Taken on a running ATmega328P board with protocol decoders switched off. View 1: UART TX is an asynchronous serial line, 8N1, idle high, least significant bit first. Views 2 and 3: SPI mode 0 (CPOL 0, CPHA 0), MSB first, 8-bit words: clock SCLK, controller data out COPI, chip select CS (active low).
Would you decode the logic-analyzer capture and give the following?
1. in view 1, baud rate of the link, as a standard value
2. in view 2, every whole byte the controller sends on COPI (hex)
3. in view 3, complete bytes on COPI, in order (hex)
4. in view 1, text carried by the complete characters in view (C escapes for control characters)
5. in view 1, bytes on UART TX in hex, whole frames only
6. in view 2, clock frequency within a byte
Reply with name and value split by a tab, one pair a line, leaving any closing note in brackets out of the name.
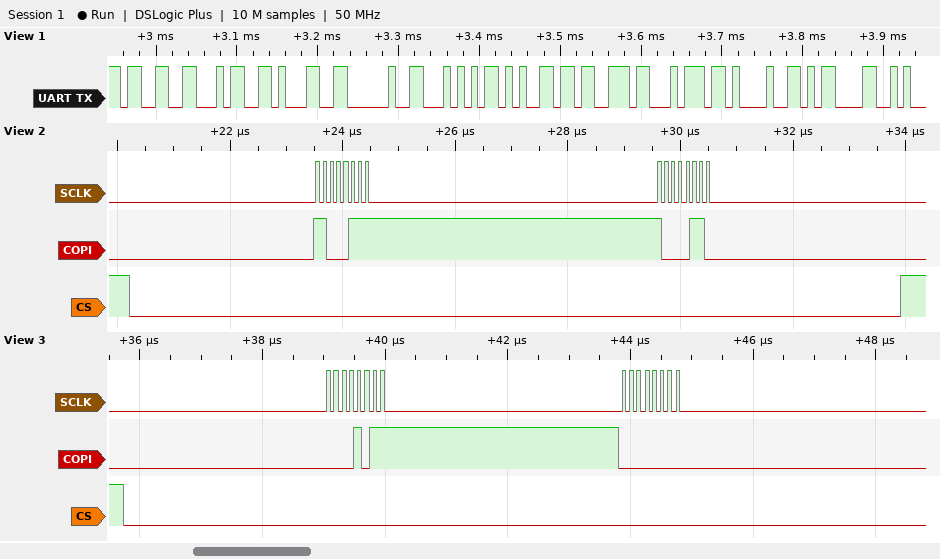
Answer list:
in view 1, baud rate of the link, as a standard value	115200 baud
in view 2, every whole byte the controller sends on COPI	C7 86
in view 3, complete bytes on COPI, in order	0B 00
in view 1, text carried by the complete characters in view	"341 Test!\r"
in view 1, bytes on UART TX in hex, whole frames only	0x33 0x34 0x31 0x20 0x54 0x65 0x73 0x74 0x21 0x0D
in view 2, clock frequency within a byte	8 MHz
